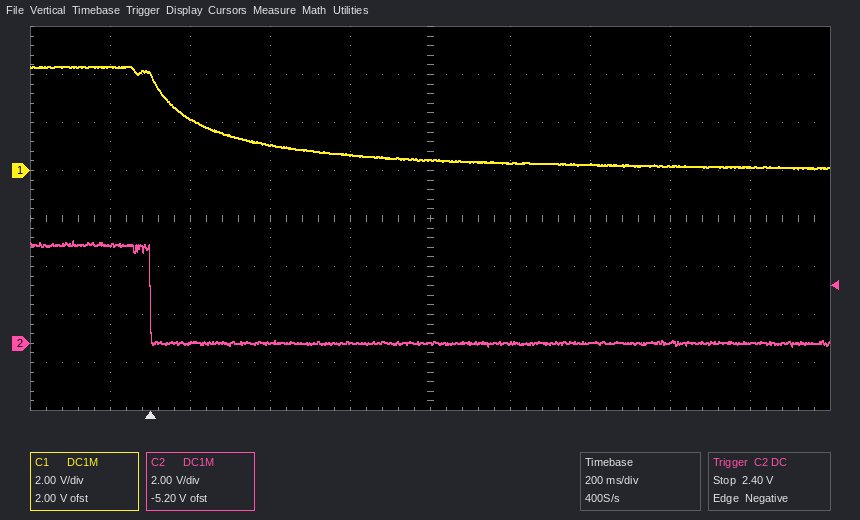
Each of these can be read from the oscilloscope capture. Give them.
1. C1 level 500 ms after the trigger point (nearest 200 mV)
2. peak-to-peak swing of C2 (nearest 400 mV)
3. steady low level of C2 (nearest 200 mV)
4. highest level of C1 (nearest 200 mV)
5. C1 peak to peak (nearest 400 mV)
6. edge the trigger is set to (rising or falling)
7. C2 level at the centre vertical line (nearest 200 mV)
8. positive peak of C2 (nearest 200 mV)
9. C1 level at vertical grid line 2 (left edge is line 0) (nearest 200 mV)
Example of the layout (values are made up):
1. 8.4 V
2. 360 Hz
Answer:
1. 600 mV
2. 4.4 V
3. 0.0 V
4. 4.4 V
5. 4.4 V
6. falling
7. 0.0 V
8. 4.2 V
9. 2.2 V
